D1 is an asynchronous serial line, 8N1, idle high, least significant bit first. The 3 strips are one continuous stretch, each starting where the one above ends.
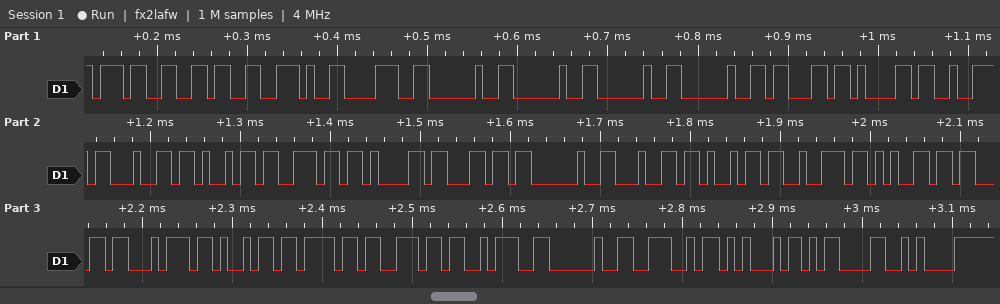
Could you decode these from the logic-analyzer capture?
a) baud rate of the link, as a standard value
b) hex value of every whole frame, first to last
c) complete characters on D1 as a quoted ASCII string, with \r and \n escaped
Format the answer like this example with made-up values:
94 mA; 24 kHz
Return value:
115200 baud; 0x37 0x36 0x2E 0x38 0x20 0x20 0x20 0x20 0x63 0x61 0x72 0x64 0x69 0x6E 0x61 0x6C 0x20 0x64 0x69 0x72 0x65 0x63 0x74 0x69 0x6F 0x6E 0x3A 0x20 0x4E 0x45 0x0D 0x0A; "76.8    cardinal direction: NE\r\n"
